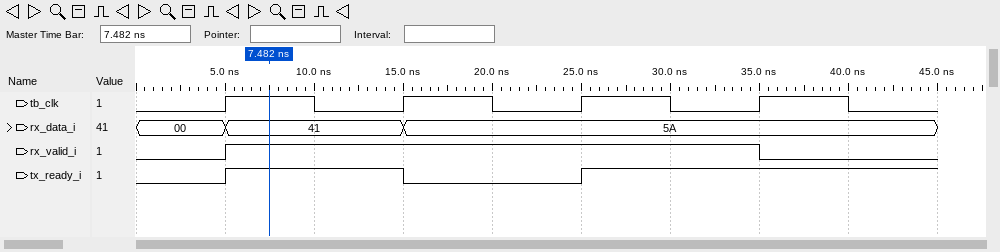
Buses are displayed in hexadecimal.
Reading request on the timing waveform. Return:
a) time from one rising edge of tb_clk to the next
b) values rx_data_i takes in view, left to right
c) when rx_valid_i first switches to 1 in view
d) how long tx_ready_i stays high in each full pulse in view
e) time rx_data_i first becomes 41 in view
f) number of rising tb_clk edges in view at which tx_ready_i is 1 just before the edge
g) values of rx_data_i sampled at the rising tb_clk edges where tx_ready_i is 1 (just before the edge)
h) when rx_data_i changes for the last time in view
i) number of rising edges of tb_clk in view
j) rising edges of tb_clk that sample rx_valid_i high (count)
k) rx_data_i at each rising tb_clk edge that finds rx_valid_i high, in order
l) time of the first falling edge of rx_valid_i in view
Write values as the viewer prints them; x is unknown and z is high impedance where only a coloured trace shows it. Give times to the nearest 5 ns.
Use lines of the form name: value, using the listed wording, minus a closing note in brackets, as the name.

time from one rising edge of tb_clk to the next: 10 ns
values rx_data_i takes in view, left to right: 00, 41, 5A
when rx_valid_i first switches to 1 in view: 5 ns
how long tx_ready_i stays high in each full pulse in view: 10 ns
time rx_data_i first becomes 41 in view: 5 ns
number of rising tb_clk edges in view at which tx_ready_i is 1 just before the edge: 2
values of rx_data_i sampled at the rising tb_clk edges where tx_ready_i is 1: 41, 5A
when rx_data_i changes for the last time in view: 15 ns
number of rising edges of tb_clk in view: 4
rising edges of tb_clk that sample rx_valid_i high: 3
rx_data_i at each rising tb_clk edge that finds rx_valid_i high, in order: 41, 5A, 5A
time of the first falling edge of rx_valid_i in view: 35 ns
